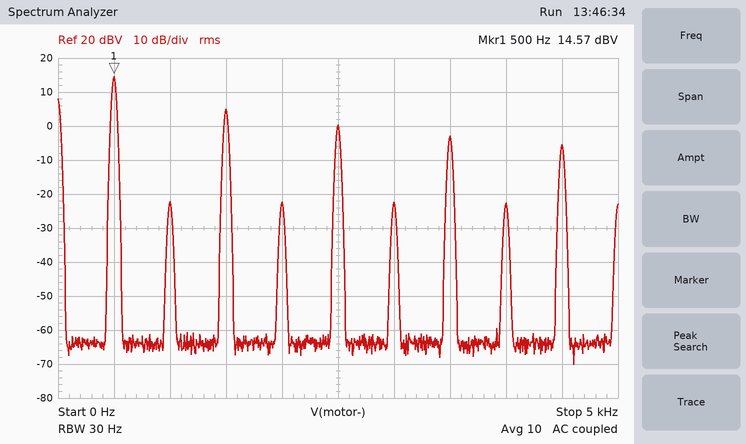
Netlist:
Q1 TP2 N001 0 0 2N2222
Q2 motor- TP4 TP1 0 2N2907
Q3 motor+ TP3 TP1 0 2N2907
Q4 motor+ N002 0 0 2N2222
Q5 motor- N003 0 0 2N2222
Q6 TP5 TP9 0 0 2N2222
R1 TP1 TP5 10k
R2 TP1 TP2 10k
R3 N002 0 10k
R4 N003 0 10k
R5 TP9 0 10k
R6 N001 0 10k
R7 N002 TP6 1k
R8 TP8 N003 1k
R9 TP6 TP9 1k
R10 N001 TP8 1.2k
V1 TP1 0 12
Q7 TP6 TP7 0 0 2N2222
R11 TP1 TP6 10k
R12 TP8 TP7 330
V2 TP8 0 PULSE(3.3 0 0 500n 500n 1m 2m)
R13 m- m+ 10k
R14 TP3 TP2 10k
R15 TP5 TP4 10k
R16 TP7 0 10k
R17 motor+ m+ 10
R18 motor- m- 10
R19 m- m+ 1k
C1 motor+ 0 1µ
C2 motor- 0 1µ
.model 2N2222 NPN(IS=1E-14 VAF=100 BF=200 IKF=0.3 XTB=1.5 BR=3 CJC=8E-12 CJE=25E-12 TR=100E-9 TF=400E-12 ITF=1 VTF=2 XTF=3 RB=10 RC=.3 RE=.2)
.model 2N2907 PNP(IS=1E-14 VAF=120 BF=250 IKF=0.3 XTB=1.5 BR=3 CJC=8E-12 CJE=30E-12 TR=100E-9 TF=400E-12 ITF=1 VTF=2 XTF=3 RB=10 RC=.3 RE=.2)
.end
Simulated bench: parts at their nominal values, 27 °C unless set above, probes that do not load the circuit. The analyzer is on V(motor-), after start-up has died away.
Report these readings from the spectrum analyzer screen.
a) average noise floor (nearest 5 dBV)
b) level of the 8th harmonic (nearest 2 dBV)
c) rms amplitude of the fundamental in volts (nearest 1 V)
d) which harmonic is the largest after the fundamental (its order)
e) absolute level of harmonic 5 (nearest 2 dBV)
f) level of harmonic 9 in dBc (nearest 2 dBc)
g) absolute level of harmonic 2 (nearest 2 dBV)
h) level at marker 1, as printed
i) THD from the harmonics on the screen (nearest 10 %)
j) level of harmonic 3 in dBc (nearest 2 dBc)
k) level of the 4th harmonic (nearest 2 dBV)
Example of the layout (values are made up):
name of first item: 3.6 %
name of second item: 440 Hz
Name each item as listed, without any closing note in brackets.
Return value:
average noise floor: -65 dBV
level of the 8th harmonic: -22 dBV
rms amplitude of the fundamental in volts: 5 V
which harmonic is the largest after the fundamental: 3
absolute level of harmonic 5: 0 dBV
level of harmonic 9 in dBc: -20 dBc
absolute level of harmonic 2: -22 dBV
level at marker 1, as printed: 14.57 dBV
THD from the harmonics on the screen: 40 %
level of harmonic 3 in dBc: -10 dBc
level of the 4th harmonic: -22 dBV
